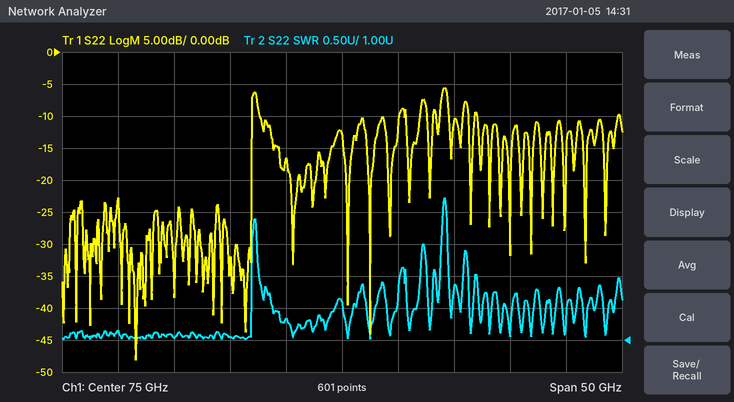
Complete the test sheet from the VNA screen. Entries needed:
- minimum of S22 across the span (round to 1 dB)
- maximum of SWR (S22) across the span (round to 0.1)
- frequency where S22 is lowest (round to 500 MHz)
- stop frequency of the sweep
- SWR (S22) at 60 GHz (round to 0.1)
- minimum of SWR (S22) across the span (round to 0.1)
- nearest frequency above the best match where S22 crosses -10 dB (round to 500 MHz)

-48 dB
3.2
56.5 GHz
100 GHz
1.0
1.0
67.0 GHz
